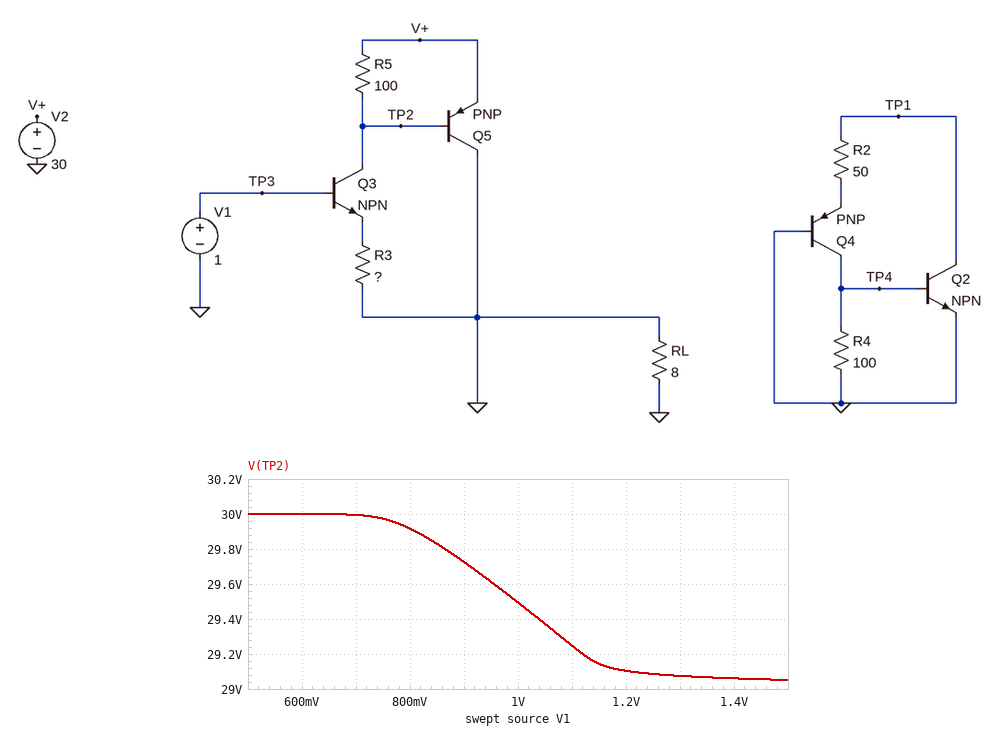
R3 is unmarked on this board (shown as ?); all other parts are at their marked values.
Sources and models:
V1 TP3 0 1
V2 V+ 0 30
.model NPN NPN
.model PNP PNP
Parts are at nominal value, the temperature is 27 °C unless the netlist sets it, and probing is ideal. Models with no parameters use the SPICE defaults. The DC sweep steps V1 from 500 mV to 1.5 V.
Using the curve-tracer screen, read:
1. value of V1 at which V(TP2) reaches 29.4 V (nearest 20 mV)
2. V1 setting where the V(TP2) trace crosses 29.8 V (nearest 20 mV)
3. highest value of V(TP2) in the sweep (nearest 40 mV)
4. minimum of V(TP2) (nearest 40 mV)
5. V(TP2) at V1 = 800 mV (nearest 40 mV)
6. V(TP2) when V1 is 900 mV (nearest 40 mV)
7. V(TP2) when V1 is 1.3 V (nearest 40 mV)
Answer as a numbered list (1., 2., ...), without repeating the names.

1. 1.04 V
2. 860 mV
3. 30.00 V
4. 29.04 V
5. 29.92 V
6. 29.72 V
7. 29.08 V
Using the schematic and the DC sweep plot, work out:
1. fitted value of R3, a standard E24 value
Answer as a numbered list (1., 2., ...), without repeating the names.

1. 36 Ω
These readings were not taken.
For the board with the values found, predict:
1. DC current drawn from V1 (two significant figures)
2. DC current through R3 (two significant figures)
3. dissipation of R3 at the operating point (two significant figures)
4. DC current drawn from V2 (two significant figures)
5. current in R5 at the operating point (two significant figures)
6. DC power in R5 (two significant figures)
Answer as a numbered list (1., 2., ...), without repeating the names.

1. 51 µA
2. 5.1 mA
3. 940 µW
4. 5.1 mA
5. 5.1 mA
6. 2.6 mW
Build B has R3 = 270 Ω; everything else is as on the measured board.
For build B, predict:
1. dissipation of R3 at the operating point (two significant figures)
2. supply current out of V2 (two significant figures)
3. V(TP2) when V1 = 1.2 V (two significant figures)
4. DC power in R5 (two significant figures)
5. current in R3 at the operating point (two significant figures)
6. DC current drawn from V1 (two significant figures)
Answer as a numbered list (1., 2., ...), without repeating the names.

1. 200 µW
2. 840 µA
3. 30 V
4. 71 µW
5. 850 µA
6. 8.4 µA
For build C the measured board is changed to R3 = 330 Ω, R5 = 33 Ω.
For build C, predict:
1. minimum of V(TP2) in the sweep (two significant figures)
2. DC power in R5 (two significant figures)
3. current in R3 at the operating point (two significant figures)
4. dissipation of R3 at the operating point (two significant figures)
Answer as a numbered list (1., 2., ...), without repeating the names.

1. 30 V
2. 16 µW
3. 710 µA
4. 170 µW
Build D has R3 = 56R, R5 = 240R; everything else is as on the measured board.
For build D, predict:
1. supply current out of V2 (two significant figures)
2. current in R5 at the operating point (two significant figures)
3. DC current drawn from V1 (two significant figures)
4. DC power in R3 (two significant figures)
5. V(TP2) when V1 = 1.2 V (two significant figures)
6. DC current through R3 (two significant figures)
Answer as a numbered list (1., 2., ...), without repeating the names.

1. 7.8 mA
2. 3.4 mA
3. 34 µA
4. 670 µW
5. 29 V
6. 3.5 mA
